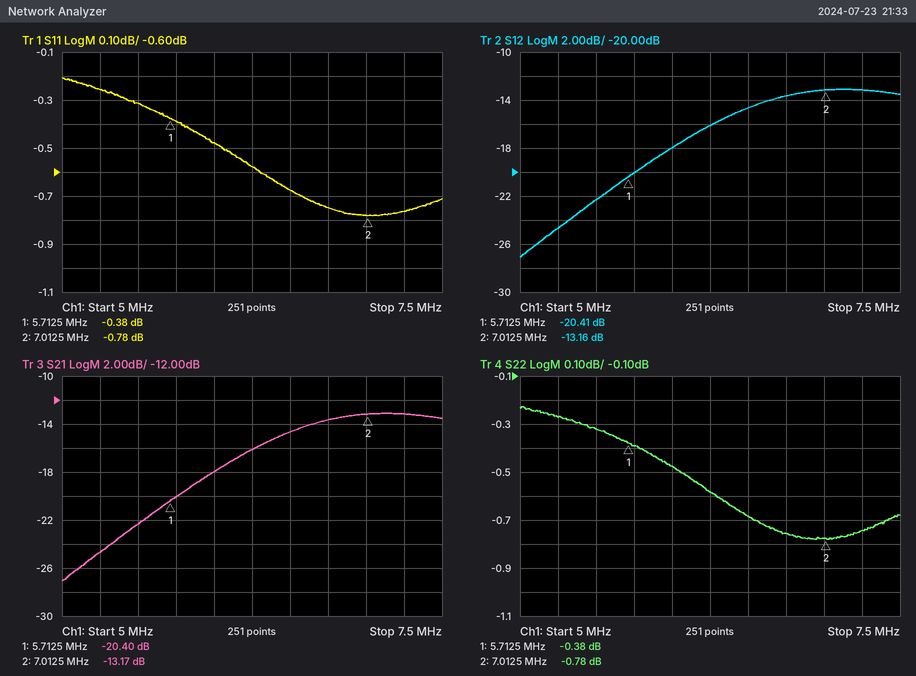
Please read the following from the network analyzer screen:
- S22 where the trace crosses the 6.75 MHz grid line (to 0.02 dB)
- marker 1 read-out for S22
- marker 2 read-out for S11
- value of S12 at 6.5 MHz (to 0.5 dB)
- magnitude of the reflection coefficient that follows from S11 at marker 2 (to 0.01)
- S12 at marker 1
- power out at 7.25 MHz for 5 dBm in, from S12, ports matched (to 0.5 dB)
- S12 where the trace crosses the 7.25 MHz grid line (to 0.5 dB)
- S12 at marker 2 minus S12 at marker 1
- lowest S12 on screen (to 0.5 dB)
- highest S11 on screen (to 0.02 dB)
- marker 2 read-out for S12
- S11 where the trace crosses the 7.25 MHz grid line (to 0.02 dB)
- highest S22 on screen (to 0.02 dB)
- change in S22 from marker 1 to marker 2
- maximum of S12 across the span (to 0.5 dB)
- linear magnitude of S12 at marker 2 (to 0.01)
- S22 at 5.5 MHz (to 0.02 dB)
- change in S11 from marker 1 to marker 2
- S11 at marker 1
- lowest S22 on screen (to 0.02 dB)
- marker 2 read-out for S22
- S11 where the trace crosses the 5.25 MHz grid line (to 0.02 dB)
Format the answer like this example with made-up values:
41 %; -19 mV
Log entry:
-0.76 dB; -0.38 dB; -0.78 dB; -14.5 dB; 0.91; -20.41 dB; -8.0 dBm; -13.0 dB; 7.25 dB; -27.0 dB; -0.20 dB; -13.16 dB; -0.76 dB; -0.22 dB; -0.40 dB; -13.0 dB; 0.22; -0.32 dB; -0.40 dB; -0.38 dB; -0.78 dB; -0.78 dB; -0.26 dB
